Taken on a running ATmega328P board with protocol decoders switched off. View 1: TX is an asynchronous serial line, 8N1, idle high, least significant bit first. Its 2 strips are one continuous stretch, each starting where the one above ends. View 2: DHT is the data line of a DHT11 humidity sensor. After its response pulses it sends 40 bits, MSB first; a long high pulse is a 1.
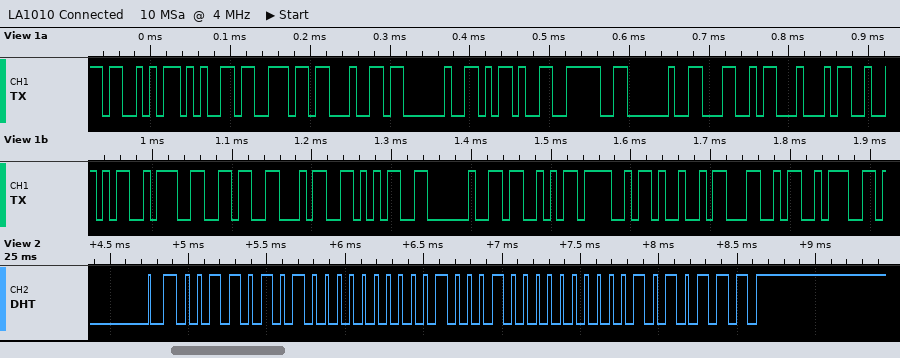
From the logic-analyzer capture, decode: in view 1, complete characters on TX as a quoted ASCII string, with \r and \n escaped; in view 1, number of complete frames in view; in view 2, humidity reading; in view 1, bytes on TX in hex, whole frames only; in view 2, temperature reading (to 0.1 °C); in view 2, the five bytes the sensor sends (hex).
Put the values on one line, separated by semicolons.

"Send -> LDR:645 SOIL:"; 21; 53 %; 53 65 6E 64 20 2D 3E 20 4C 44 52 3A 36 34 35 20 53 4F 49 4C 3A; 34.0 °C; 35 00 22 00 57
